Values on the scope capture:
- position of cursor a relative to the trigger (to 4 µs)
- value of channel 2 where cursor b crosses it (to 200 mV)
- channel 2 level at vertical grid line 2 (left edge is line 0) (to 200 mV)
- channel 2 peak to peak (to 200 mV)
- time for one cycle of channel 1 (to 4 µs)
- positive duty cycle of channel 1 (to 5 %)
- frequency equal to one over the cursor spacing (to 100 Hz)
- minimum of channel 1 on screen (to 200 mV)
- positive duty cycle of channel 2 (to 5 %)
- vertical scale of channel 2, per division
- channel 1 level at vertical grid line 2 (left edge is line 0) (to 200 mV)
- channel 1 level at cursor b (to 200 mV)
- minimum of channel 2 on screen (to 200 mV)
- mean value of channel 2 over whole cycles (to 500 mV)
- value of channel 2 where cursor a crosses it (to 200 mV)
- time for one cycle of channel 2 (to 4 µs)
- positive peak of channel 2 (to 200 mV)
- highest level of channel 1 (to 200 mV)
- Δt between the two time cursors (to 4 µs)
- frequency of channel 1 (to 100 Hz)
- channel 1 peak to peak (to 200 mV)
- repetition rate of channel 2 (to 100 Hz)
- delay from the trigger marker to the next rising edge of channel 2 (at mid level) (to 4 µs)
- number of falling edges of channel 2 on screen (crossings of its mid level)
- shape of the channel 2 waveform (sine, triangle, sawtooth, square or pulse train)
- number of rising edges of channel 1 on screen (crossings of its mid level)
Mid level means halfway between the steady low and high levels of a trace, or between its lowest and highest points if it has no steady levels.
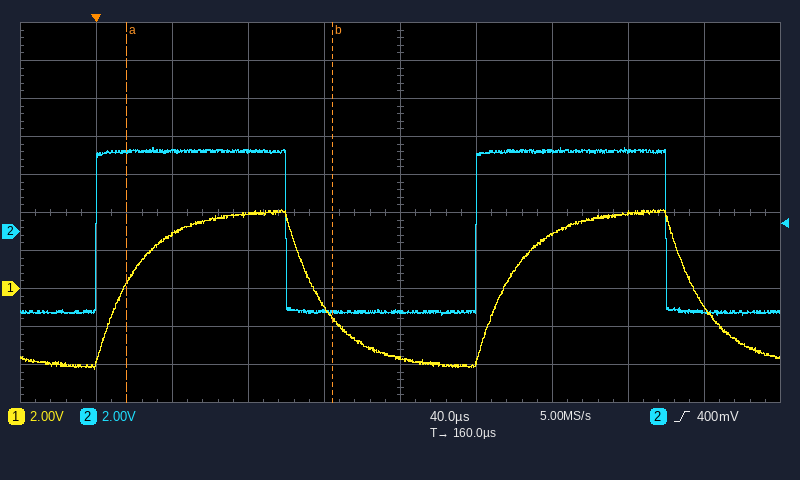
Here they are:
+16 µs
-4.2 V
4.2 V
8.8 V
200 µs
50 %
9.3 kHz
-4.2 V
50 %
2 V
2.8 V
-1.6 V
-4.4 V
0.0 V
4.2 V
200 µs
4.4 V
4.2 V
108 µs
5.0 kHz
8.4 V
5.0 kHz
200 µs
2
square
2
